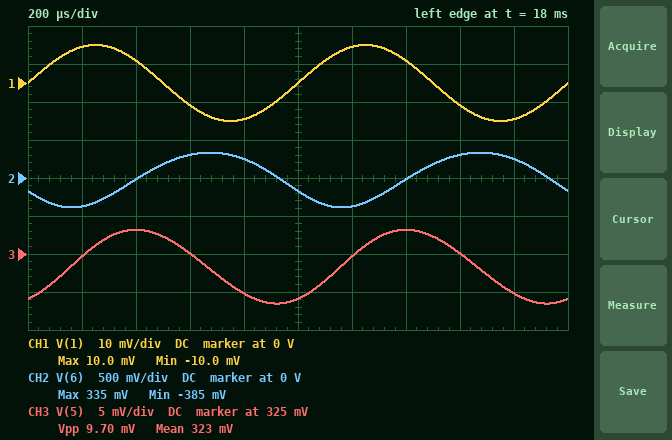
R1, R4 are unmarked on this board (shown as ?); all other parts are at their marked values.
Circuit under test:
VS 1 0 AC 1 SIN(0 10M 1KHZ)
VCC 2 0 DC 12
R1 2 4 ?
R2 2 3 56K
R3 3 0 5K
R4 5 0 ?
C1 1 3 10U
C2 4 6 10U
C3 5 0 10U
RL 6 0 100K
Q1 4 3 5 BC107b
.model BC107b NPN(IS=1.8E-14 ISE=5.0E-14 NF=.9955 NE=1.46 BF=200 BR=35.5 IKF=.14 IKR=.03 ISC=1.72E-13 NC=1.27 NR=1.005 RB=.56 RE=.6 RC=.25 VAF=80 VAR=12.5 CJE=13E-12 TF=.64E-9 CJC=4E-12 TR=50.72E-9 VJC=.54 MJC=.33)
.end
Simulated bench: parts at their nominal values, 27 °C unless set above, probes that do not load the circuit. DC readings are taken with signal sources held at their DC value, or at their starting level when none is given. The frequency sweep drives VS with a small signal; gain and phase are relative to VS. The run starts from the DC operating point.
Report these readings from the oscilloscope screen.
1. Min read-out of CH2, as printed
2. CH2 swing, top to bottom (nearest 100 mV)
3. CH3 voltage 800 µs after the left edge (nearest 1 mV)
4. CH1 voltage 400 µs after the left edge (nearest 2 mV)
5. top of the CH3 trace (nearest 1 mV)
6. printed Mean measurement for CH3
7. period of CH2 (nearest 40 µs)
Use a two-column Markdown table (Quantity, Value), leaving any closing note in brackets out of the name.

| Quantity | Value |
|---|---|
| Min read-out of CH2, as printed | -385 mV |
| CH2 swing, top to bottom | 700 mV |
| CH3 voltage 800 µs after the left edge | 320 mV |
| CH1 voltage 400 µs after the left edge | 6 mV |
| top of the CH3 trace | 328 mV |
| printed Mean measurement for CH3 | 323 mV |
| period of CH2 | 1.00 ms |
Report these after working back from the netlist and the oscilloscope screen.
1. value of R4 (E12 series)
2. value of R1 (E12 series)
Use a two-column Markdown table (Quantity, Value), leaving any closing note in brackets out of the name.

| Quantity | Value |
|---|---|
| value of R4 | 330 Ω |
| value of R1 | 1.2 kΩ |
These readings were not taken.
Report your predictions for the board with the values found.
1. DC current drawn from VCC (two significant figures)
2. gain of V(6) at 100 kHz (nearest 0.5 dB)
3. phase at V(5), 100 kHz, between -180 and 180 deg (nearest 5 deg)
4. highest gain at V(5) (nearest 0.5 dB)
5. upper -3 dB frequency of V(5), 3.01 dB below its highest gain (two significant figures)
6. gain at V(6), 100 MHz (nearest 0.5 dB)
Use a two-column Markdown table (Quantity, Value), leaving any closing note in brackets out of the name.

| Quantity | Value |
|---|---|
| DC current drawn from VCC | 1.2 mA |
| gain of V(6) at 100 kHz | 32.5 dB |
| phase at V(5), 100 kHz, between -180 and 180 deg | -90 deg |
| highest gain at V(5) | -1.0 dB |
| upper -3 dB frequency of V(5), 3.01 dB below its highest gain | 640 Hz |
| gain at V(6), 100 MHz | 29.0 dB |
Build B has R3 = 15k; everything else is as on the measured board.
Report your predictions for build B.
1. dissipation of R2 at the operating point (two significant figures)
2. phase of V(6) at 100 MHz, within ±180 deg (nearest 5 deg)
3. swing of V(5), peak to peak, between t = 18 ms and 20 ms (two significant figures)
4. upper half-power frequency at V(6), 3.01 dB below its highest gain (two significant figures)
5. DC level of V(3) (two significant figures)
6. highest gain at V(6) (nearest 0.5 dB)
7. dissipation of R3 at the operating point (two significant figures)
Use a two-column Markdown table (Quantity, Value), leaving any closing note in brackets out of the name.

| Quantity | Value |
|---|---|
| dissipation of R2 at the operating point | 1.7 mW |
| phase of V(6) at 100 MHz, within ±180 deg | 120 deg |
| swing of V(5), peak to peak, between t = 18 ms and 20 ms | 18 mV |
| upper half-power frequency at V(6), 3.01 dB below its highest gain | 67 MHz |
| DC level of V(3) | 2.2 V |
| highest gain at V(6) | 45.0 dB |
| dissipation of R3 at the operating point | 330 µW |
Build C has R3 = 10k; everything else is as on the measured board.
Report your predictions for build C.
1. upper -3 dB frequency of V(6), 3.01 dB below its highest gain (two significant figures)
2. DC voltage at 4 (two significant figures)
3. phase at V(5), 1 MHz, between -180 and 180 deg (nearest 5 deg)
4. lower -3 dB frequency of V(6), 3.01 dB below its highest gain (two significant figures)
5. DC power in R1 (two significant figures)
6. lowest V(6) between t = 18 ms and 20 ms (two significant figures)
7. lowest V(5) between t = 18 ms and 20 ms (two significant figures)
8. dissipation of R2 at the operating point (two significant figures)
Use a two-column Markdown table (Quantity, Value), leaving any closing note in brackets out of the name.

| Quantity | Value |
|---|---|
| upper -3 dB frequency of V(6), 3.01 dB below its highest gain | 77 MHz |
| DC voltage at 4 | 8.4 V |
| phase at V(5), 1 MHz, between -180 and 180 deg | -90 deg |
| lower -3 dB frequency of V(6), 3.01 dB below its highest gain | 1.7 kHz |
| DC power in R1 | 11 mW |
| lowest V(6) between t = 18 ms and 20 ms | -630 mV |
| lowest V(5) between t = 18 ms and 20 ms | 1.0 V |
| dissipation of R2 at the operating point | 1.9 mW |
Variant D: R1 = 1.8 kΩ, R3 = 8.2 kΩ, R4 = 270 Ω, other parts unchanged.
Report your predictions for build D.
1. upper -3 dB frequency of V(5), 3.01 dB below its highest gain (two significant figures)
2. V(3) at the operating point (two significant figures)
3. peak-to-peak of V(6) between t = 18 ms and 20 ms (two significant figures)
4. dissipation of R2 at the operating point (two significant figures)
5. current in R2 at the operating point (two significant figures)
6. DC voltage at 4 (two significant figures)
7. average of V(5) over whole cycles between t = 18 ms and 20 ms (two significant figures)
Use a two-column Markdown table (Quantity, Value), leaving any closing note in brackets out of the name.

| Quantity | Value |
|---|---|
| upper -3 dB frequency of V(5), 3.01 dB below its highest gain | 1.6 kHz |
| V(3) at the operating point | 1.4 V |
| peak-to-peak of V(6) between t = 18 ms and 20 ms | 1.8 V |
| dissipation of R2 at the operating point | 2.0 mW |
| current in R2 at the operating point | 190 µA |
| DC voltage at 4 | 7.0 V |
| average of V(5) over whole cycles between t = 18 ms and 20 ms | 750 mV |
